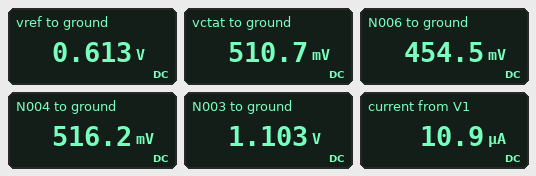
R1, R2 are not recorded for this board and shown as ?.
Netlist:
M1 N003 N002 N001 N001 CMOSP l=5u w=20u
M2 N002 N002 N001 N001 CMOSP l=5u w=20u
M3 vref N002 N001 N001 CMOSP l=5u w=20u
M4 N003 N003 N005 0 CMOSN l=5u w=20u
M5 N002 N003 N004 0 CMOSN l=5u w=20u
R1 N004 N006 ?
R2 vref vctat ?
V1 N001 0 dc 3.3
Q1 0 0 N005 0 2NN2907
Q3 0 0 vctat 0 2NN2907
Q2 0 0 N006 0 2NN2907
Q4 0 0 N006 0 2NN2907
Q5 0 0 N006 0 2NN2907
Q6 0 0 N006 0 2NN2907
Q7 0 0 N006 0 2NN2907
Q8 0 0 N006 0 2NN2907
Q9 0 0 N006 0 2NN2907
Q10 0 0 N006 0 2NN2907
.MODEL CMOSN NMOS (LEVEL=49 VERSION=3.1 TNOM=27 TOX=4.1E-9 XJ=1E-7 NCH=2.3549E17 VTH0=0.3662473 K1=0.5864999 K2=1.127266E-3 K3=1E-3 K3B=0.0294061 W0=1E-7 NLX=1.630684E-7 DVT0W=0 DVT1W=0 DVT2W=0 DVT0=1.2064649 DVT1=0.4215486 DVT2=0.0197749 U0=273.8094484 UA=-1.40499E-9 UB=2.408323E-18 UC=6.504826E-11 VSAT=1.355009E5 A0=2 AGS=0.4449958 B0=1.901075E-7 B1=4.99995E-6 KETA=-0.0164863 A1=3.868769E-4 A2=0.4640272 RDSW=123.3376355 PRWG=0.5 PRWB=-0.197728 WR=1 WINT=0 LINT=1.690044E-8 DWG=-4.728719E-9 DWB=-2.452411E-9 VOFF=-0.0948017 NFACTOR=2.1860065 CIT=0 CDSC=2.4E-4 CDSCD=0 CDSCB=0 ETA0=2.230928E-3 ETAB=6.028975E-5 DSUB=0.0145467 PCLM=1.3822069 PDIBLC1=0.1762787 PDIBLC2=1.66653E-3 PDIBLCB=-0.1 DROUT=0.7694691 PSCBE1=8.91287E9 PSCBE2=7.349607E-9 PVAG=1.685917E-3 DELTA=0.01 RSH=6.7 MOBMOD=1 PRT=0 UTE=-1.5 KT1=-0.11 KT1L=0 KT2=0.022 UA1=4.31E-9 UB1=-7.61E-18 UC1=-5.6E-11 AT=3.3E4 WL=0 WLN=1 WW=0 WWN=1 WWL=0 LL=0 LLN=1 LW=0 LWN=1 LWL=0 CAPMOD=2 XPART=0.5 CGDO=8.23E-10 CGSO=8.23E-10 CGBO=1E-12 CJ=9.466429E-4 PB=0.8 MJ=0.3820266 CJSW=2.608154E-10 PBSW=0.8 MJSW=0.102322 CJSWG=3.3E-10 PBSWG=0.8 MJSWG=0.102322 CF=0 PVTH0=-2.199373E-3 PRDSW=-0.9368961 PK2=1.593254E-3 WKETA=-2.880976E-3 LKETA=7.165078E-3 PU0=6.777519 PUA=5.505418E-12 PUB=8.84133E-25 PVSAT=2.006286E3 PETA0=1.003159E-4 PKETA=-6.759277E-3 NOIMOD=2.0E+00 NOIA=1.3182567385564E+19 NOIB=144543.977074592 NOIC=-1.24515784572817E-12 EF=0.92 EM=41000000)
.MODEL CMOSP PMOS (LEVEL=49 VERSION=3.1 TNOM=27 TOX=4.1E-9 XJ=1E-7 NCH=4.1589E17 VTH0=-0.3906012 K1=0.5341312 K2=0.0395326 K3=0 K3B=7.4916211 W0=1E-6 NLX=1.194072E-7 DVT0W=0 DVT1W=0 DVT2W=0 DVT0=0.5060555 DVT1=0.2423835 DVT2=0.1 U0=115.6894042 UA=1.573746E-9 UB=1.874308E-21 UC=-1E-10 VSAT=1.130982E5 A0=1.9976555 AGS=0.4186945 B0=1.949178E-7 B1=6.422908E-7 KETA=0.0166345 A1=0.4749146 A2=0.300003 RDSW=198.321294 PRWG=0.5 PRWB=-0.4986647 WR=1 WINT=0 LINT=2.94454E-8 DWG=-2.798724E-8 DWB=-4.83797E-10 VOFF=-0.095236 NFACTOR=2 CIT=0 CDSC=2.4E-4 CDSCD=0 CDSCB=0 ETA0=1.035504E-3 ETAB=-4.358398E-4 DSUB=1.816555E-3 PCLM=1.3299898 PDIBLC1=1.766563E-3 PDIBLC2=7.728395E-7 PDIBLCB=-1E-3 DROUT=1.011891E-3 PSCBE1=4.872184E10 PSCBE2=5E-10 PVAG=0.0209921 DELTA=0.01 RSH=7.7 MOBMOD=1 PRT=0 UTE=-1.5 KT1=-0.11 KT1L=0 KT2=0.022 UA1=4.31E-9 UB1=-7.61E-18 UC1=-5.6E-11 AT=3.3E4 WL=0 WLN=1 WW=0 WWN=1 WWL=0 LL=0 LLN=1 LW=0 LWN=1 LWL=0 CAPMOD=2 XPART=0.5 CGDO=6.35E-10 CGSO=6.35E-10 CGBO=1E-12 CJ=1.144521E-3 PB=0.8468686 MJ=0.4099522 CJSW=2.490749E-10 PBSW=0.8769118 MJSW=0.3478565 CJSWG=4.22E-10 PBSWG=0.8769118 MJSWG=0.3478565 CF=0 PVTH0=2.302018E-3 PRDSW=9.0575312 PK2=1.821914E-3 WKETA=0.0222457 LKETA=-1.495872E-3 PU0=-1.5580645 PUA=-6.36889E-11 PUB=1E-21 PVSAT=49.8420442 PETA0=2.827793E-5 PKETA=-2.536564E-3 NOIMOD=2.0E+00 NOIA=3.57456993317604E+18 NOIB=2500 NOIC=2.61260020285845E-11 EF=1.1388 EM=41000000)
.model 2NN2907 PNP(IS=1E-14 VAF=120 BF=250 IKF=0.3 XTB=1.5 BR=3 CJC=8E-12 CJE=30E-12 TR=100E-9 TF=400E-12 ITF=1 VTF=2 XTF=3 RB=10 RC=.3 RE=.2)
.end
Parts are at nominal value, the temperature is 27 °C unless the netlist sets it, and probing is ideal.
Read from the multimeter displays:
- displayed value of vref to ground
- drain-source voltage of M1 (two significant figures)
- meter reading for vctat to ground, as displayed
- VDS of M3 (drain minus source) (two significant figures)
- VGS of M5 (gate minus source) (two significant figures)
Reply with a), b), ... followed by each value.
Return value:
a) 0.613 V
b) -2.2 V
c) 510.7 mV
d) -2.7 V
e) 590 mV
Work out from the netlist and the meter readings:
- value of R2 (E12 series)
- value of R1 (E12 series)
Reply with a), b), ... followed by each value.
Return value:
a) 27 kΩ
b) 18 kΩ
